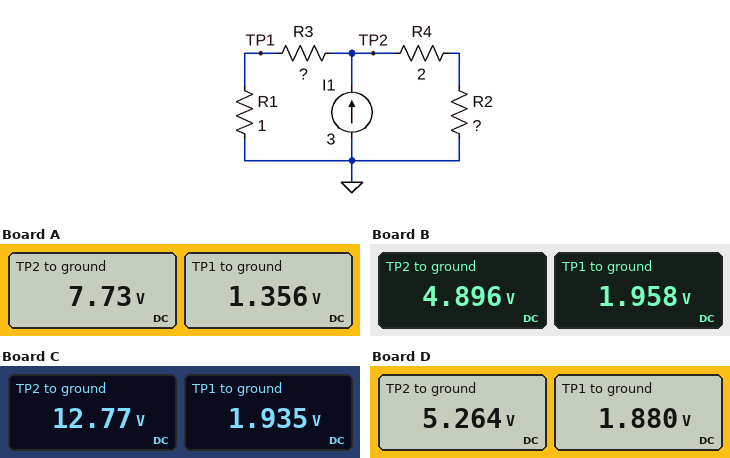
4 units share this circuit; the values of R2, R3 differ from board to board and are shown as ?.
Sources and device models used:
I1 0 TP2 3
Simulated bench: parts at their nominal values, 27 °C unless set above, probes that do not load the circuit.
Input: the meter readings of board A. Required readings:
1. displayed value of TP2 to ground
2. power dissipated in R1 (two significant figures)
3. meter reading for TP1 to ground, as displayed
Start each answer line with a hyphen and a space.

- 7.73 V
- 1.8 W
- 1.356 V
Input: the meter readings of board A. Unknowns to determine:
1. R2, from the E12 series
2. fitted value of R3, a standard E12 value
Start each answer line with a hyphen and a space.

- 2.7 Ω
- 4.7 Ω
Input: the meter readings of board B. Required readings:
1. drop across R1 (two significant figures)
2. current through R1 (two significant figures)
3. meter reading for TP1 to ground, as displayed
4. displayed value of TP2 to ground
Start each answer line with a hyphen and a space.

- 2.0 V
- 2.0 A
- 1.958 V
- 4.896 V
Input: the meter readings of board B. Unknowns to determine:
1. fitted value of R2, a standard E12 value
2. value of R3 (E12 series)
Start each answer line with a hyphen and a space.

- 2.7 Ω
- 1.5 Ω
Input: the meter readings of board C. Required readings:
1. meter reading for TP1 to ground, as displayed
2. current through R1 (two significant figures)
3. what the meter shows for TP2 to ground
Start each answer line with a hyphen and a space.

- 1.935 V
- 1.9 A
- 12.77 V
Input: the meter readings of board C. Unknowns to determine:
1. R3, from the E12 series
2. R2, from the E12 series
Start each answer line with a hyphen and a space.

- 5.6 Ω
- 10 Ω
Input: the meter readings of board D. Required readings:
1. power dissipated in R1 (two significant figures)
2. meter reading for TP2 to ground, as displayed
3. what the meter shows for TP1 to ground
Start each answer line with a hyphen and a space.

- 3.5 W
- 5.264 V
- 1.880 V
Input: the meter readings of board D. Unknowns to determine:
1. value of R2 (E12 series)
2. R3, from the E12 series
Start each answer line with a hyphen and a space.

- 2.7 Ω
- 1.8 Ω
